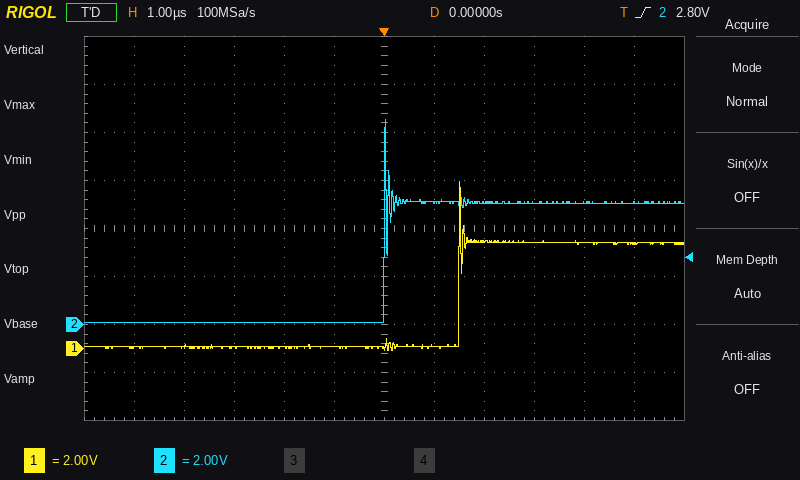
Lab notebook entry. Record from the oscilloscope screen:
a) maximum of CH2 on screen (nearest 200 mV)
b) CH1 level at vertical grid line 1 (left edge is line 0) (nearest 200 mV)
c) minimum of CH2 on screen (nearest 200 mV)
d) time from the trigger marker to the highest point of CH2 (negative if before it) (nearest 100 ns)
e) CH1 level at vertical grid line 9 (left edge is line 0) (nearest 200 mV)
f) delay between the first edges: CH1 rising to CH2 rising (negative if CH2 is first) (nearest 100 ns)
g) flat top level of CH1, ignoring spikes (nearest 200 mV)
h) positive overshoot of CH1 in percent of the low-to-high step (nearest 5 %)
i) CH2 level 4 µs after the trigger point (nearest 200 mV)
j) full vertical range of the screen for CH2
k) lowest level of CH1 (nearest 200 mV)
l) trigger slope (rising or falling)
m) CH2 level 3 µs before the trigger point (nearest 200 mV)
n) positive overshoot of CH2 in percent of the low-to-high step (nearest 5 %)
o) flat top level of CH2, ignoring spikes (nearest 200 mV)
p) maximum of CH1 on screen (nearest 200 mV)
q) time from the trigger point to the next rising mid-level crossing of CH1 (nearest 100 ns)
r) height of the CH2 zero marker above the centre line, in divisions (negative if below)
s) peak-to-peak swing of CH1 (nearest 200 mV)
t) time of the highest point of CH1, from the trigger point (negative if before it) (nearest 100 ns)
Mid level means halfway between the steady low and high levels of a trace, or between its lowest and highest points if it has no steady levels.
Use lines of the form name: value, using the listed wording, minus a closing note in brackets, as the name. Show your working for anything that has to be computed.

maximum of CH2 on screen: 8.6 V
CH1 level at vertical grid line 1 (left edge is line 0): 0.0 V
minimum of CH2 on screen: 0.0 V
time from the trigger marker to the highest point of CH2 (negative if before it): 0.0 µs
CH1 level at vertical grid line 9 (left edge is line 0): 4.4 V
delay between the first edges: CH1 rising to CH2 rising (negative if CH2 is first): -1.5 µs
flat top level of CH1, ignoring spikes: 4.4 V
positive overshoot of CH1 in percent of the low-to-high step: 60 %
CH2 level 4 µs after the trigger point: 5.0 V
full vertical range of the screen for CH2: 16 V
lowest level of CH1: 0.0 V
trigger slope: rising
CH2 level 3 µs before the trigger point: 0.0 V
positive overshoot of CH2 in percent of the low-to-high step: 70 %
flat top level of CH2, ignoring spikes: 5.0 V
maximum of CH1 on screen: 7.0 V
time from the trigger point to the next rising mid-level crossing of CH1: 1.5 µs
height of the CH2 zero marker above the centre line, in divisions: -2.0 div
peak-to-peak swing of CH1: 7.0 V − (0.0 V) = 7.0 V
time of the highest point of CH1, from the trigger point (negative if before it): +1.5 µs
